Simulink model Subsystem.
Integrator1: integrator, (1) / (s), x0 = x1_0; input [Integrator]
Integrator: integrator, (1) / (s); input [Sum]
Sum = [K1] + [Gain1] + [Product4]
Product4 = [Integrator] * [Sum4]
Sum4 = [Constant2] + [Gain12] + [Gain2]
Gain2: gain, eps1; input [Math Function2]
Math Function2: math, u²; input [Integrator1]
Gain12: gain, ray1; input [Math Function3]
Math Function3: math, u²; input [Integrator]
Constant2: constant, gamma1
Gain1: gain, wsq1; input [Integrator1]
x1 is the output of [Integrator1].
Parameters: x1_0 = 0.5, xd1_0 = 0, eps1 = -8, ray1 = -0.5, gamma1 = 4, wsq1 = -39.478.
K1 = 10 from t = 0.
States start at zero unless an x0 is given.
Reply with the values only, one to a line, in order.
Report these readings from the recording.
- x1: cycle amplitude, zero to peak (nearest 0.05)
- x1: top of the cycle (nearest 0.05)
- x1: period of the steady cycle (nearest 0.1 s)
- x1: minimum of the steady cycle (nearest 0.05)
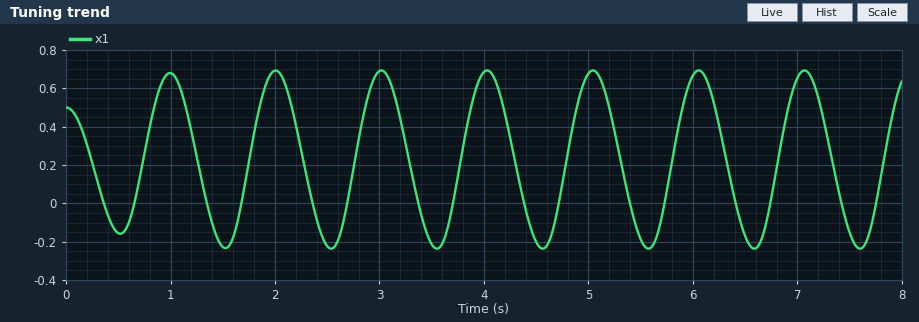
0.45
0.70
1.0 s
-0.25
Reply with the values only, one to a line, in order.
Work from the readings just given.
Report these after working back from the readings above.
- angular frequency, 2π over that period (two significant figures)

6.3 rad/s
